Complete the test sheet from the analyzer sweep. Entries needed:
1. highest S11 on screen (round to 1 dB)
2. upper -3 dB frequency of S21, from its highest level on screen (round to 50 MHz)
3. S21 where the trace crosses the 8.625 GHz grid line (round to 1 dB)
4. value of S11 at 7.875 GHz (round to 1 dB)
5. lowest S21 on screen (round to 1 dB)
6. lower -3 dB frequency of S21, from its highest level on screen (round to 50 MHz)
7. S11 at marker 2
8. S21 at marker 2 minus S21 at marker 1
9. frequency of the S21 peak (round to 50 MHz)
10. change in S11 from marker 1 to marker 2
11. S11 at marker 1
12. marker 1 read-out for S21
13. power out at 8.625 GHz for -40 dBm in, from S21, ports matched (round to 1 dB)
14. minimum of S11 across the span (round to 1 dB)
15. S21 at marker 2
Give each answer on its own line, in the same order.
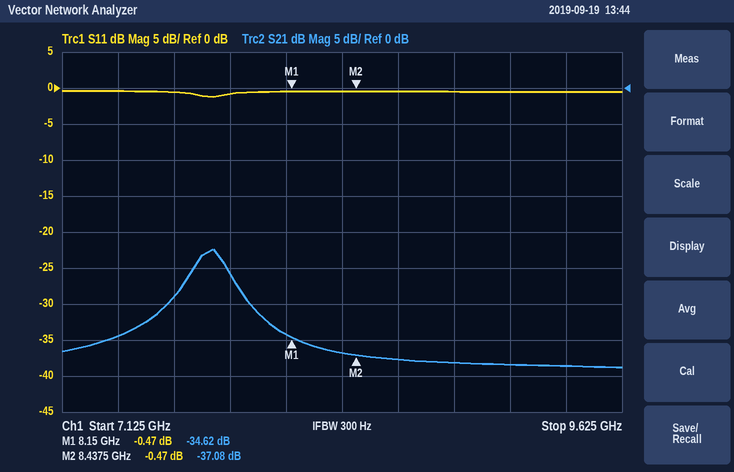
0 dB
7.85 GHz
-38 dB
-1 dB
-39 dB
7.70 GHz
-0.47 dB
-2.46 dB
7.80 GHz
0.00 dB
-0.47 dB
-34.62 dB
-78 dBm
-1 dB
-37.08 dB
